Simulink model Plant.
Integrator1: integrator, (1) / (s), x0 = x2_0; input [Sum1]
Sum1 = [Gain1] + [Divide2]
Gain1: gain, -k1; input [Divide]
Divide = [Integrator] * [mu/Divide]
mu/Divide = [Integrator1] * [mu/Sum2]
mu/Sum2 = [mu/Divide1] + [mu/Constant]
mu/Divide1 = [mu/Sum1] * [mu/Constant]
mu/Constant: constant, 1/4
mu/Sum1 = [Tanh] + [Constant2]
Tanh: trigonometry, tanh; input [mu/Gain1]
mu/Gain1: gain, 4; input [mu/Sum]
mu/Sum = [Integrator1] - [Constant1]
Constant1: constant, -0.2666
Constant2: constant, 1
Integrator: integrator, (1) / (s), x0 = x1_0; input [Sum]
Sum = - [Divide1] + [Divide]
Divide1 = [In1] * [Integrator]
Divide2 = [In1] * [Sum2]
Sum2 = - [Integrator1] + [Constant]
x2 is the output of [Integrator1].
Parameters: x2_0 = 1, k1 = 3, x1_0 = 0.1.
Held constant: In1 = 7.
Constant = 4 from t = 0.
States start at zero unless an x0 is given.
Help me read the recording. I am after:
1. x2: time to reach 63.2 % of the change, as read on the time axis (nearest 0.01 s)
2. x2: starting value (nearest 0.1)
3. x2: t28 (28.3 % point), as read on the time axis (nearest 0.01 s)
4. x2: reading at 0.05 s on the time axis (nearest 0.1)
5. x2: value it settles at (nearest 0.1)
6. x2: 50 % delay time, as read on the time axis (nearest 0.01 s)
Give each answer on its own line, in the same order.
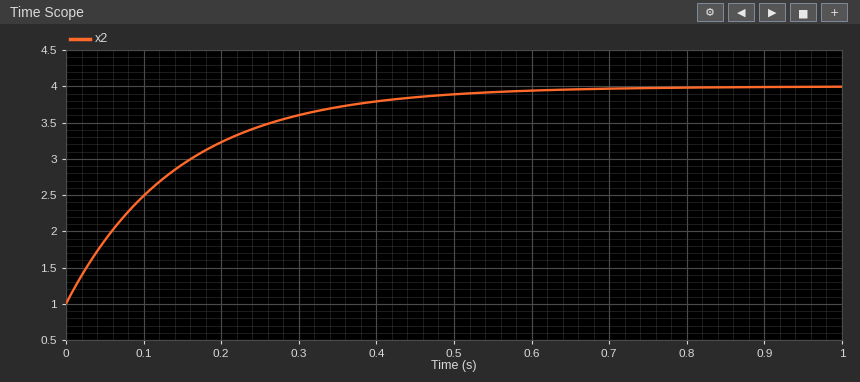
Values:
0.15 s
1.0
0.05 s
1.9
4.0
0.10 s
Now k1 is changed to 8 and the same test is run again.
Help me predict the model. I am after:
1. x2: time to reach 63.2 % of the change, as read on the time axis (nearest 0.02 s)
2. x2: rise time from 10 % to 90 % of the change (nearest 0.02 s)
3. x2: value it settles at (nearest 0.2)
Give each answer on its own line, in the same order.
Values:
0.16 s
0.36 s
4.0
